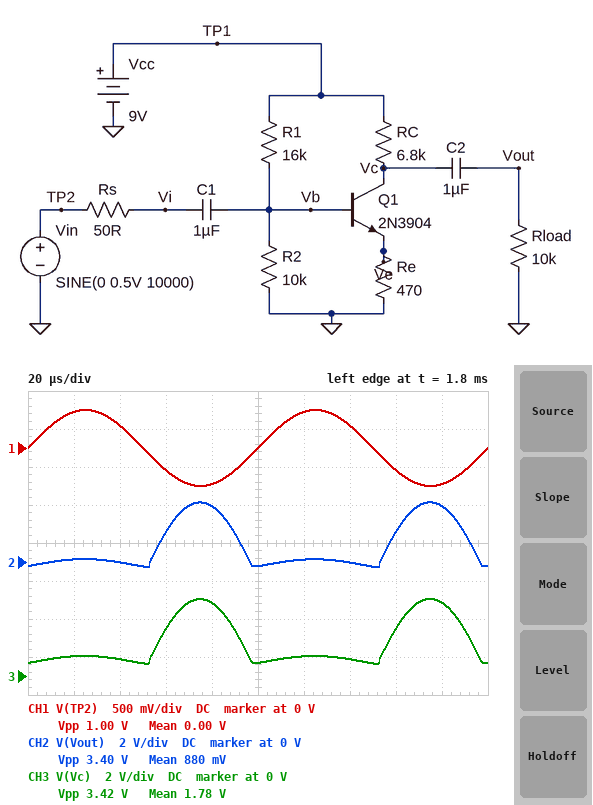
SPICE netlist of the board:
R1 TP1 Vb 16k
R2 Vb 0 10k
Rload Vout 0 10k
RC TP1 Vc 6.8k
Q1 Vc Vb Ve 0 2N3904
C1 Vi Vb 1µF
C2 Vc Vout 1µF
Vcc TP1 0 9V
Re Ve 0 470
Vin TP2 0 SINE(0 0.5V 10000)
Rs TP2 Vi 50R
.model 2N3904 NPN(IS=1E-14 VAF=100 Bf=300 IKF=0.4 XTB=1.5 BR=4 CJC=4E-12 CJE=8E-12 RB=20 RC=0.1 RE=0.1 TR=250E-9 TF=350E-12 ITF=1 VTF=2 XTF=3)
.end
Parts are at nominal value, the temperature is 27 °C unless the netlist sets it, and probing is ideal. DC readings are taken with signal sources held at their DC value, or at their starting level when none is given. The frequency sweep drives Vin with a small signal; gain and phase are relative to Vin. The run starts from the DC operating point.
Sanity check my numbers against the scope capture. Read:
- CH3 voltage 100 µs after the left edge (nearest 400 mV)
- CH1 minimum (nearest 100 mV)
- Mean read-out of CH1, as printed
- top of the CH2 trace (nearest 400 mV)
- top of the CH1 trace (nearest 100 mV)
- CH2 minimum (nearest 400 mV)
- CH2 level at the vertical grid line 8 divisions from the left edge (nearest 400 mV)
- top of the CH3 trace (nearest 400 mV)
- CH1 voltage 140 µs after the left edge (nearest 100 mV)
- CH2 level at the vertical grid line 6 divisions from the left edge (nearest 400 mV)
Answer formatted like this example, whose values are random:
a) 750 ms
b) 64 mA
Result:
a) 800 mV
b) -500 mV
c) 0.00 V
d) 3.2 V
e) 500 mV
f) -400 mV
g) 1.6 V
h) 4.0 V
i) 300 mV
j) 0 V
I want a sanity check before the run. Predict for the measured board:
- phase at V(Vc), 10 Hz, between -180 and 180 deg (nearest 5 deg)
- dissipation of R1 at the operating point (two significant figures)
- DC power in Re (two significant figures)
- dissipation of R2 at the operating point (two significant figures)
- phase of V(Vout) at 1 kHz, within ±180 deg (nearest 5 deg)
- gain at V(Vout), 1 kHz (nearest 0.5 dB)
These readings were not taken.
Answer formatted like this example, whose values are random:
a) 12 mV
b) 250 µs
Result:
a) 85 deg
b) 3.6 mW
c) 1.1 mW
d) 200 µW
e) 20 deg
f) -3.5 dB
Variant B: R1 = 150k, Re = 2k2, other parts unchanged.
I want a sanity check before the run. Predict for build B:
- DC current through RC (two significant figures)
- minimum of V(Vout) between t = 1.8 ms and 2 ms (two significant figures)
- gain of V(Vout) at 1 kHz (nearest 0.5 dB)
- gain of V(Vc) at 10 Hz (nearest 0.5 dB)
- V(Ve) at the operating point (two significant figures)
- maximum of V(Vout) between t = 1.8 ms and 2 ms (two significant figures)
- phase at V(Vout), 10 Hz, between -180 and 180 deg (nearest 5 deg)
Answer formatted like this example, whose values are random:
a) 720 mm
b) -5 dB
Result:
a) 11 µA
b) -750 mV
c) -1.0 dB
d) -4.0 dB
e) 25 mV
f) 70 mV
g) -75 deg
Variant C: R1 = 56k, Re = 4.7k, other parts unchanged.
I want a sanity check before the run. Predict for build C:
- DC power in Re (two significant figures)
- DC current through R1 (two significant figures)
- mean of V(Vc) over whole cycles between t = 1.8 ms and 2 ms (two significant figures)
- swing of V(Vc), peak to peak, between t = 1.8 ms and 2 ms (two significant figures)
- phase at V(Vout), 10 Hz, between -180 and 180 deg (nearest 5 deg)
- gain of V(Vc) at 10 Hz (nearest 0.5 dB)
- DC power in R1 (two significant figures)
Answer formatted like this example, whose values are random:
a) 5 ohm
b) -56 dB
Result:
a) 120 µW
b) 140 µA
c) 7.9 V
d) 820 mV
e) -75 deg
f) -5.5 dB
g) 1.0 mW
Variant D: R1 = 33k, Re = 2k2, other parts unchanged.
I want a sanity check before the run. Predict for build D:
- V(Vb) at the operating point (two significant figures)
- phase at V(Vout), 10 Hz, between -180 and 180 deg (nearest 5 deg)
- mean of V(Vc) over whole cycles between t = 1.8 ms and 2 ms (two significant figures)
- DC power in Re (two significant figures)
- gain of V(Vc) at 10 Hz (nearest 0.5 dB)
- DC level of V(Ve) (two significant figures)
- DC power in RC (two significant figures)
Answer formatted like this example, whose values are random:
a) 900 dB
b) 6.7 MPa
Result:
a) 2.1 V
b) -70 deg
c) 4.6 V
d) 930 µW
e) 0.5 dB
f) 1.4 V
g) 2.9 mW
